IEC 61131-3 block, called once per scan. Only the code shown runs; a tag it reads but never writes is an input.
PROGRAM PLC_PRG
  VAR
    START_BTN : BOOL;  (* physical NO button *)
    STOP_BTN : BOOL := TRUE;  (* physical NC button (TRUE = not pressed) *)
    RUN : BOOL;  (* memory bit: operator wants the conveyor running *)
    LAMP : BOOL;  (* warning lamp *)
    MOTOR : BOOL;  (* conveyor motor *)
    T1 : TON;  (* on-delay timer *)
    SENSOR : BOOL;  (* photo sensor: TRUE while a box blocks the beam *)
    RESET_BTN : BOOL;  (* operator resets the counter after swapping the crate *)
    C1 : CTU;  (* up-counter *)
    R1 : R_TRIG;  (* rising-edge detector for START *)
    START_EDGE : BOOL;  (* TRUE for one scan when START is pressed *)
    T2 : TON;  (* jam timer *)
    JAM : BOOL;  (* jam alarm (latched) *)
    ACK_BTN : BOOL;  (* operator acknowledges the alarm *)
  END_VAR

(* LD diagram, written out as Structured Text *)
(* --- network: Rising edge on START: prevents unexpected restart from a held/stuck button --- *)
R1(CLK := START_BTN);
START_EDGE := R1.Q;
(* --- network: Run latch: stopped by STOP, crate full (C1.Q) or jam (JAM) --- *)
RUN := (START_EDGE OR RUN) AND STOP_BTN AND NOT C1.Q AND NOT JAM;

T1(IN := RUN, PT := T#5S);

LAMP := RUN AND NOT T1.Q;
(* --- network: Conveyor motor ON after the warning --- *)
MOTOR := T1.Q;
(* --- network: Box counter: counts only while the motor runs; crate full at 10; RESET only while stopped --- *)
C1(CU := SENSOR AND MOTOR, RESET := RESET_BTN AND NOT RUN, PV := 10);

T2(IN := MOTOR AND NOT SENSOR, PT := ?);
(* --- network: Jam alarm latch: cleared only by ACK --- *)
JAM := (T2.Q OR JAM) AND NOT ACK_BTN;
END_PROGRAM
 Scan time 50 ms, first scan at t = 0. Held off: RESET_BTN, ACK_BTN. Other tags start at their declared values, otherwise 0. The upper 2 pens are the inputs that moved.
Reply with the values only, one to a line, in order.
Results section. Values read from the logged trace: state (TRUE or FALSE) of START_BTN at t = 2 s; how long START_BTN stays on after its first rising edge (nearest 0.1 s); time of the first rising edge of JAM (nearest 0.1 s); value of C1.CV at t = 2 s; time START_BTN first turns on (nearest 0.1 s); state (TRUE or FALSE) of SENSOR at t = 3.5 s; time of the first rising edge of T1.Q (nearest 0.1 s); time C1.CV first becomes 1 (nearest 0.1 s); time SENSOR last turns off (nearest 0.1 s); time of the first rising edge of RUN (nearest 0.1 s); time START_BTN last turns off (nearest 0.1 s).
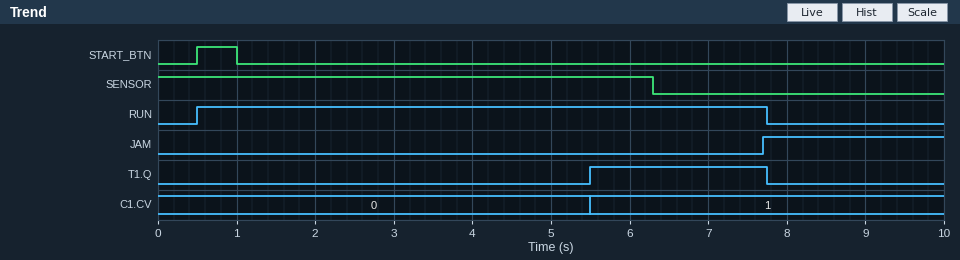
FALSE
0.5 s
7.7 s
0
0.5 s
TRUE
5.5 s
5.5 s
6.3 s
0.5 s
1.0 s
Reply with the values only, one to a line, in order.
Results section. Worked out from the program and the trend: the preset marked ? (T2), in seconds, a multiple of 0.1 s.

1.4 s
